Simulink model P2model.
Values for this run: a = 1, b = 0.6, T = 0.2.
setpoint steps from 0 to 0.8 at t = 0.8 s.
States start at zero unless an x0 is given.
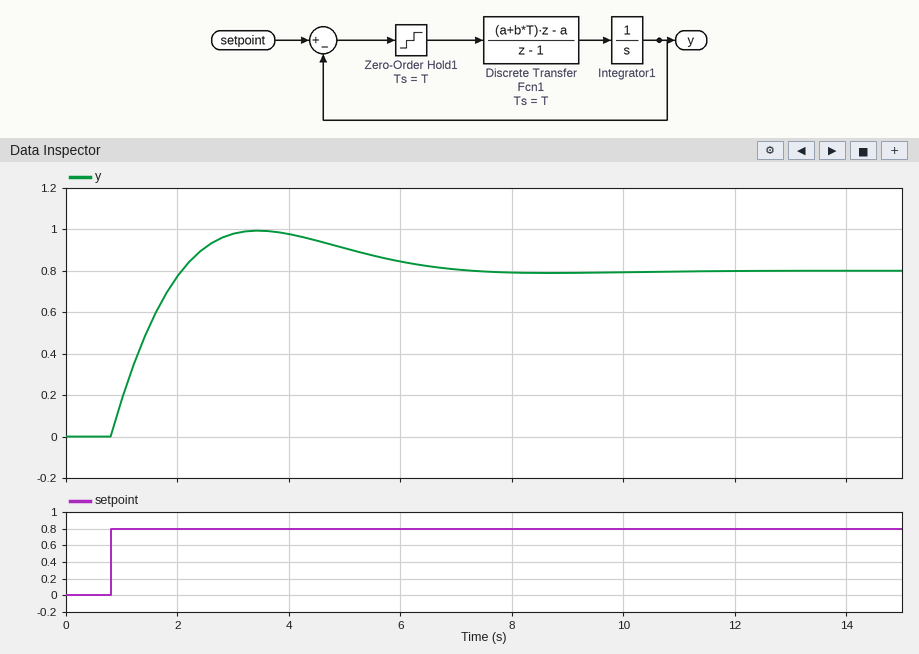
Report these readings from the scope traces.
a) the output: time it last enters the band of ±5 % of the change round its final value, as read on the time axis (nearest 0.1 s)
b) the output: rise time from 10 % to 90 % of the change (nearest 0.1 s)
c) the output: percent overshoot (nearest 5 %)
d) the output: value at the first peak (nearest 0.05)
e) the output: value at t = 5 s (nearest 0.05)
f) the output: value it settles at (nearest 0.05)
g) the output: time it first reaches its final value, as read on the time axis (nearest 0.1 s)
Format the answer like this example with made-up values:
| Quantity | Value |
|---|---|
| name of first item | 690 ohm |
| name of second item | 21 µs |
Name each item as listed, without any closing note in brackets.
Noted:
| Quantity | Value |
|---|---|
| the output: time it last enters the band of ±5 % of the change round its final value, as read on the time axis | 6.1 s |
| the output: rise time from 10 % to 90 % of the change | 1.0 s |
| the output: percent overshoot | 25 % |
| the output: value at the first peak | 1.00 |
| the output: value at t = 5 s | 0.90 |
| the output: value it settles at | 0.80 |
| the output: time it first reaches its final value, as read on the time axis | 2.1 s |
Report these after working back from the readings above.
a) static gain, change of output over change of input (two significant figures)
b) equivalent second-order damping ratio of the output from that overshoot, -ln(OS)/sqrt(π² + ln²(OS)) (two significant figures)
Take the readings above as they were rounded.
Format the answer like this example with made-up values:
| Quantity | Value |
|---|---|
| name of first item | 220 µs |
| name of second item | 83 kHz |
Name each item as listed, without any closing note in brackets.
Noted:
| Quantity | Value |
|---|---|
| static gain, change of output over change of input | 1.0 |
| equivalent second-order damping ratio of the output from that overshoot, -ln(OS)/sqrt(π² + ln²(OS)) | 0.40 |
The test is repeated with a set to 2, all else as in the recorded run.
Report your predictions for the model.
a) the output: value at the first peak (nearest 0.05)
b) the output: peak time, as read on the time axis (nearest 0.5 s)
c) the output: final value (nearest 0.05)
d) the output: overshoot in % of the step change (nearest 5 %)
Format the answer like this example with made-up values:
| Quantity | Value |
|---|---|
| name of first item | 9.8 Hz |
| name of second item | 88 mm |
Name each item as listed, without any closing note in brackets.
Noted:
| Quantity | Value |
|---|---|
| the output: value at the first peak | 0.90 |
| the output: peak time, as read on the time axis | 2.5 s |
| the output: final value | 0.80 |
| the output: overshoot in % of the step change | 10 % |
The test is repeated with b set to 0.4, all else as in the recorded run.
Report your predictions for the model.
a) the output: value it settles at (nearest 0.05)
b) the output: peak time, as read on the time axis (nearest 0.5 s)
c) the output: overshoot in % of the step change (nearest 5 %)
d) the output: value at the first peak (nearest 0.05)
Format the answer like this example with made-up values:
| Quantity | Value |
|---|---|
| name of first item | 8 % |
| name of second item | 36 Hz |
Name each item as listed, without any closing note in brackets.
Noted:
| Quantity | Value |
|---|---|
| the output: value it settles at | 0.80 |
| the output: peak time, as read on the time axis | 4.0 s |
| the output: overshoot in % of the step change | 20 % |
| the output: value at the first peak | 0.95 |
